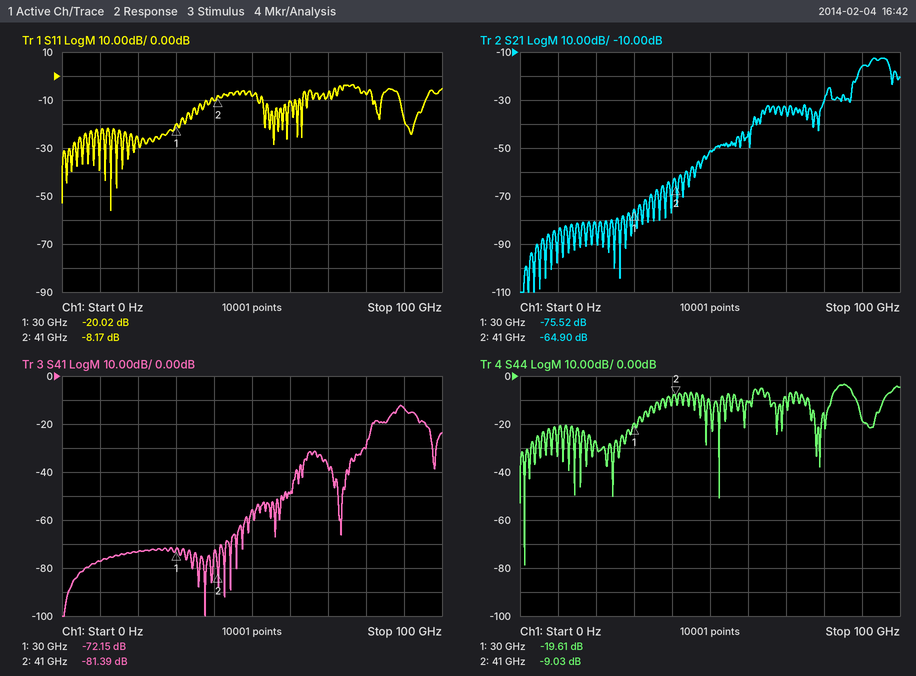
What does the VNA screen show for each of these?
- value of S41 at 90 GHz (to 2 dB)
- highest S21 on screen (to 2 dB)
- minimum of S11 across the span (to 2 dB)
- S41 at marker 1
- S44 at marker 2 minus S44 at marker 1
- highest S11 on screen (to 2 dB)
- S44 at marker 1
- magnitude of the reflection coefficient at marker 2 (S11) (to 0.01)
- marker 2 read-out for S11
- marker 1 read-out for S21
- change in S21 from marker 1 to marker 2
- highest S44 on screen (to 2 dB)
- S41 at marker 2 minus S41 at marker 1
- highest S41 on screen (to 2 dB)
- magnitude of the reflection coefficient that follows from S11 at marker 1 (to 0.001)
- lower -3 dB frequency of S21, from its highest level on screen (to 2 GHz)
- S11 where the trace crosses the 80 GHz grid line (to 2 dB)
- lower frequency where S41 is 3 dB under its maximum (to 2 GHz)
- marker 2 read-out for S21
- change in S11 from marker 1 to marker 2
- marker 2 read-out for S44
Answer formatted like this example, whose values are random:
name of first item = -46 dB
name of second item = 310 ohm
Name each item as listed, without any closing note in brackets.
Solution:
value of S41 at 90 GHz = -14 dB
highest S21 on screen = -12 dB
minimum of S11 across the span = -56 dB
S41 at marker 1 = -72.15 dB
S44 at marker 2 minus S44 at marker 1 = 10.58 dB
highest S11 on screen = -4 dB
S44 at marker 1 = -19.61 dB
magnitude of the reflection coefficient at marker 2 (S11) = 0.39
marker 2 read-out for S11 = -8.17 dB
marker 1 read-out for S21 = -75.52 dB
change in S21 from marker 1 to marker 2 = 10.62 dB
highest S44 on screen = -4 dB
S41 at marker 2 minus S41 at marker 1 = -9.24 dB
highest S41 on screen = -12 dB
magnitude of the reflection coefficient that follows from S11 at marker 1 = 0.100
lower -3 dB frequency of S21, from its highest level on screen = 92 GHz
S11 where the trace crosses the 80 GHz grid line = -8 dB
lower frequency where S41 is 3 dB under its maximum = 88 GHz
marker 2 read-out for S21 = -64.90 dB
change in S11 from marker 1 to marker 2 = 11.85 dB
marker 2 read-out for S44 = -9.03 dB
